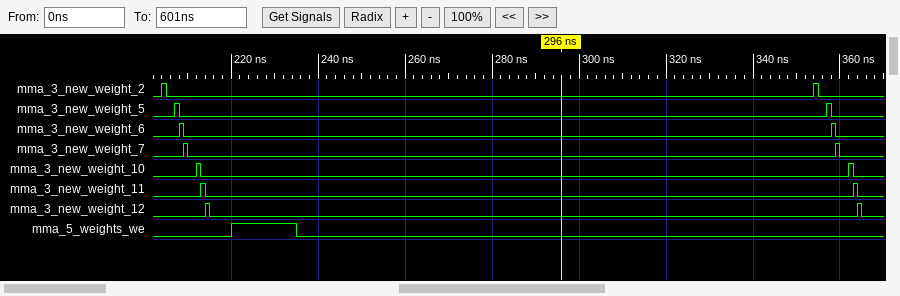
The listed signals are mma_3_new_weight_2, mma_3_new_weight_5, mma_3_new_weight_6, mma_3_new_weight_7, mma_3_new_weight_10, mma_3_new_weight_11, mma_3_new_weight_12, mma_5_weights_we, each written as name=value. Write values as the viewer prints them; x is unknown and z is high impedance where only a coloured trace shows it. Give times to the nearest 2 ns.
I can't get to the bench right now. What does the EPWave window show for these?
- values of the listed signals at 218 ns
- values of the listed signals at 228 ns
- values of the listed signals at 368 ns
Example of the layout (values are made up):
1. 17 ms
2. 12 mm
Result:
1. mma_3_new_weight_2=0, mma_3_new_weight_5=0, mma_3_new_weight_6=0, mma_3_new_weight_7=0, mma_3_new_weight_10=0, mma_3_new_weight_11=0, mma_3_new_weight_12=0, mma_5_weights_we=0
2. mma_3_new_weight_2=0, mma_3_new_weight_5=0, mma_3_new_weight_6=0, mma_3_new_weight_7=0, mma_3_new_weight_10=0, mma_3_new_weight_11=0, mma_3_new_weight_12=0, mma_5_weights_we=1
3. mma_3_new_weight_2=0, mma_3_new_weight_5=0, mma_3_new_weight_6=0, mma_3_new_weight_7=0, mma_3_new_weight_10=0, mma_3_new_weight_11=0, mma_3_new_weight_12=0, mma_5_weights_we=0
